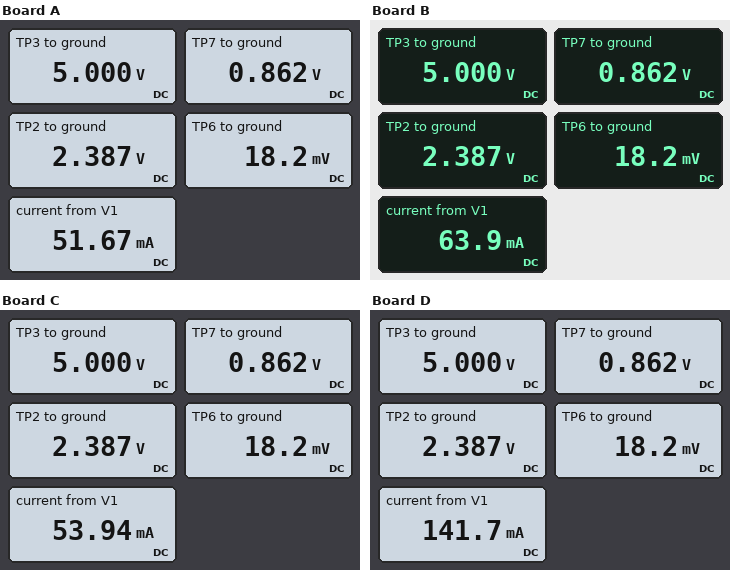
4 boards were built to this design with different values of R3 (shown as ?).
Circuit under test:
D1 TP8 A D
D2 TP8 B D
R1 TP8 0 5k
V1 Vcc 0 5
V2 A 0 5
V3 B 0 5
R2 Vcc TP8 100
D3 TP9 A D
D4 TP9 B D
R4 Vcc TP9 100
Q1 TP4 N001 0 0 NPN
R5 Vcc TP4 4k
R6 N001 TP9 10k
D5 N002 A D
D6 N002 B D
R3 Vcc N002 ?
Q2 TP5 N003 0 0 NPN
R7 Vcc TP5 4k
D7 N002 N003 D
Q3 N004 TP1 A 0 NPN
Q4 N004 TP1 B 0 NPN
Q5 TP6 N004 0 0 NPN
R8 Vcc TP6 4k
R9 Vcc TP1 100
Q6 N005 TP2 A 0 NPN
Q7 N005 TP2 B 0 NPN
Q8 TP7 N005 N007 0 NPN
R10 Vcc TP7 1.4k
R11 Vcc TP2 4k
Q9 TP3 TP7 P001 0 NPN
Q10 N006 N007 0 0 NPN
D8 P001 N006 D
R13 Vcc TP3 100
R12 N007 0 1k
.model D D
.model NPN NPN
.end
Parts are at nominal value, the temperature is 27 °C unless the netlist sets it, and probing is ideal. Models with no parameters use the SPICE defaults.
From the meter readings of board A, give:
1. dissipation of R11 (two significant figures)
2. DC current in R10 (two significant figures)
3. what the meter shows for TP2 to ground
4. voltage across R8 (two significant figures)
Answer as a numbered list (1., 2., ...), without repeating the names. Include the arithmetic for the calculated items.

1. (5 V - 2.387 V)^2 / 4 kΩ = 1.7 mW
2. (5 V - 862 mV) / 1.4 kΩ = 3.0 mA
3. 2.387 V
4. 5 V - 18.2 mV = 5.0 V
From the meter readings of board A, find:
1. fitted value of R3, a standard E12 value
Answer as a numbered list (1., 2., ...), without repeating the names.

1. 330 Ω
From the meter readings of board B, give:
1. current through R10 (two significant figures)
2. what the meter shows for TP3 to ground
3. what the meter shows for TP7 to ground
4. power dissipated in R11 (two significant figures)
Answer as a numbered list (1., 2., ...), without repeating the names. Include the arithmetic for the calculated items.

1. (5 V - 862 mV) / 1.4 kΩ = 3.0 mA
2. 5.000 V
3. 0.862 V
4. (5 V - 2.387 V)^2 / 4 kΩ = 1.7 mW
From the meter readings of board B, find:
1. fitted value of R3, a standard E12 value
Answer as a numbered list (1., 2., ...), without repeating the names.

1. 150 Ω
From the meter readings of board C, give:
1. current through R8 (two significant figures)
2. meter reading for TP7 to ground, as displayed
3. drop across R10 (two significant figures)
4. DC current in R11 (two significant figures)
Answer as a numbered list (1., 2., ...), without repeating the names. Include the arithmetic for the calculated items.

1. (5 V - 18.2 mV) / 4 kΩ = 1.2 mA
2. 0.862 V
3. 5 V - 862 mV = 4.1 V
4. (5 V - 2.387 V) / 4 kΩ = 650 µA
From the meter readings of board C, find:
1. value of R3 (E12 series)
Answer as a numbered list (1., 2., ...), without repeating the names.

1. 270 Ω
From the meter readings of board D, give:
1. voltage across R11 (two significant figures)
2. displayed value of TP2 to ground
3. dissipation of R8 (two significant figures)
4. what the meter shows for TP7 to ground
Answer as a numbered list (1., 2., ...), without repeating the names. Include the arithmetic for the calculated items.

1. 5 V - 2.387 V = 2.6 V
2. 2.387 V
3. (5 V - 18.2 mV)^2 / 4 kΩ = 6.2 mW
4. 0.862 V
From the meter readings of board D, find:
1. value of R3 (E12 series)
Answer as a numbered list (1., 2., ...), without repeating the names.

1. 33 Ω
